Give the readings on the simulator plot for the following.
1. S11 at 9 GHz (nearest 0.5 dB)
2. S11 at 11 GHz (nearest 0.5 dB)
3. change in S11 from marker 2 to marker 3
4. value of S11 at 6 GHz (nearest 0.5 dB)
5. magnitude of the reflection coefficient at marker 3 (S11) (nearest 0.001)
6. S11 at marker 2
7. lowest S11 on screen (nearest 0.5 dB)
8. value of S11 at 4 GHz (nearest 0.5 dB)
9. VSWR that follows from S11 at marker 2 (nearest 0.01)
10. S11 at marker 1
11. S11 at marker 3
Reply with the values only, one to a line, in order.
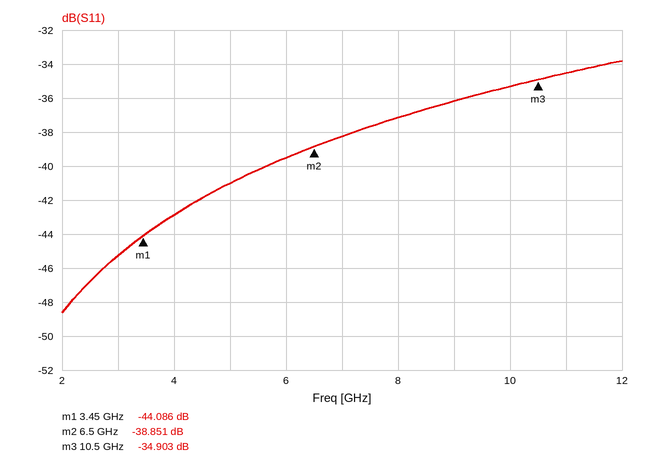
-36.0 dB
-34.5 dB
3.948 dB
-39.5 dB
0.018
-38.851 dB
-48.5 dB
-43.0 dB
1.02
-44.086 dB
-34.903 dB
